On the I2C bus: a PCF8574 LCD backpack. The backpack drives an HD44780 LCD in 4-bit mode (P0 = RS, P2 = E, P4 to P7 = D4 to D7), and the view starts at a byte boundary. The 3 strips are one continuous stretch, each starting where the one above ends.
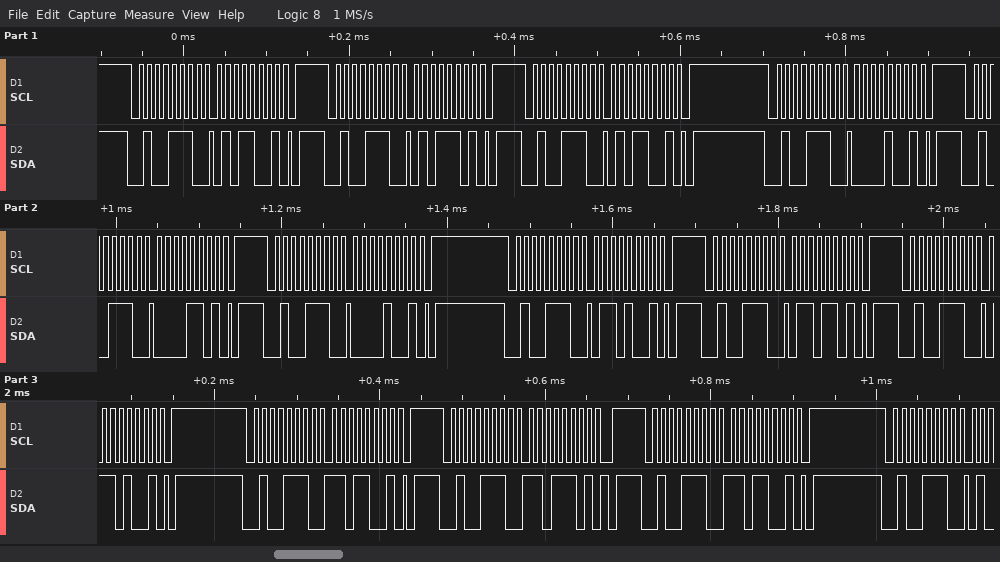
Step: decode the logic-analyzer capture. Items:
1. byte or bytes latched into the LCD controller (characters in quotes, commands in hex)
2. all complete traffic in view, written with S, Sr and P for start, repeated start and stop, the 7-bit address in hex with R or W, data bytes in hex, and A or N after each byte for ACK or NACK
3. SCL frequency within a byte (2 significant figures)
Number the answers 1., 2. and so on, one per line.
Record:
1. 'P' 'm'
2. S 27W A 59 A P S 27W A 5D A P S 27W A 59 A P S 27W A 09 A P S 27W A 0D A P S 27W A 09 A P S 27W A 69 A P S 27W A 6D A P S 27W A 69 A P S 27W A D9 A P S 27W A DD A P S 27W A D9 A P S 27W A
3. 100 kHz
